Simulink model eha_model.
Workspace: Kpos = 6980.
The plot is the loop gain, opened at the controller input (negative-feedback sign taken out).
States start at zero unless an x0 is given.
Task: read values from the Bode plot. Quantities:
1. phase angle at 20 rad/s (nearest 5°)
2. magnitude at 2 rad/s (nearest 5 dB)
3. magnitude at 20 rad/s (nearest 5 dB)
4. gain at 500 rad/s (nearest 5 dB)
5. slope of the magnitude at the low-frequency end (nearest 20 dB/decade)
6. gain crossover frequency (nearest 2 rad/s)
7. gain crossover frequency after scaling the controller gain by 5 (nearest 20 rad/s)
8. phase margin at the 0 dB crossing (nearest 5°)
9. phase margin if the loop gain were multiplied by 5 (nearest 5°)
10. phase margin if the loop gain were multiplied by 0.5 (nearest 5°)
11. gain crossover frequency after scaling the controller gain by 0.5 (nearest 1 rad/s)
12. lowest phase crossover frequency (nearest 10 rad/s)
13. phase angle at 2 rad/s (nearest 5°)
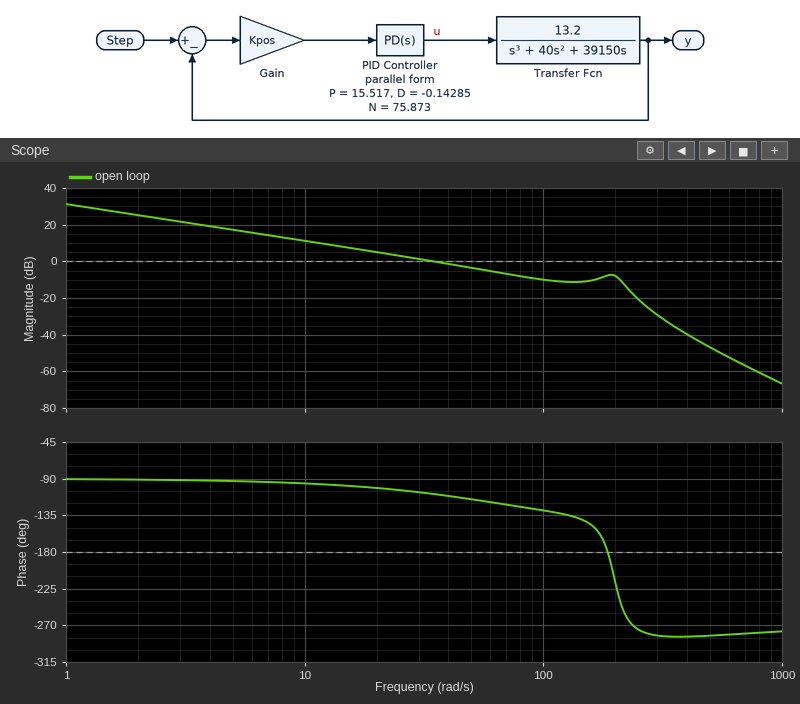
-100°
25 dB
5 dB
-45 dB
-20 dB/decade
34 rad/s
220 rad/s
70°
-80°
80°
18 rad/s
190 rad/s
-90°
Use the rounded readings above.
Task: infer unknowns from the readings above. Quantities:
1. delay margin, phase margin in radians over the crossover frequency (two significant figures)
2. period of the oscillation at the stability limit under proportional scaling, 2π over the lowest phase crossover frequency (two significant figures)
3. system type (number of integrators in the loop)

0.036 s
0.033 s
1
